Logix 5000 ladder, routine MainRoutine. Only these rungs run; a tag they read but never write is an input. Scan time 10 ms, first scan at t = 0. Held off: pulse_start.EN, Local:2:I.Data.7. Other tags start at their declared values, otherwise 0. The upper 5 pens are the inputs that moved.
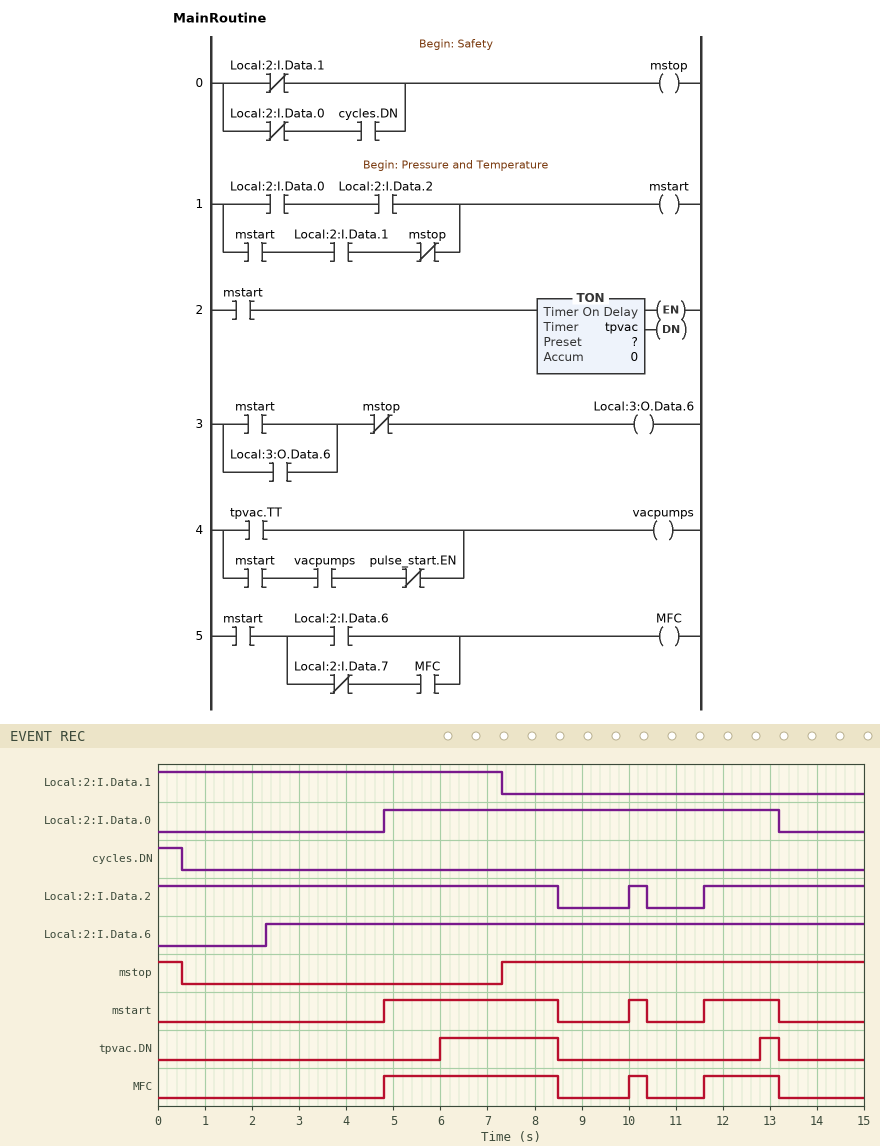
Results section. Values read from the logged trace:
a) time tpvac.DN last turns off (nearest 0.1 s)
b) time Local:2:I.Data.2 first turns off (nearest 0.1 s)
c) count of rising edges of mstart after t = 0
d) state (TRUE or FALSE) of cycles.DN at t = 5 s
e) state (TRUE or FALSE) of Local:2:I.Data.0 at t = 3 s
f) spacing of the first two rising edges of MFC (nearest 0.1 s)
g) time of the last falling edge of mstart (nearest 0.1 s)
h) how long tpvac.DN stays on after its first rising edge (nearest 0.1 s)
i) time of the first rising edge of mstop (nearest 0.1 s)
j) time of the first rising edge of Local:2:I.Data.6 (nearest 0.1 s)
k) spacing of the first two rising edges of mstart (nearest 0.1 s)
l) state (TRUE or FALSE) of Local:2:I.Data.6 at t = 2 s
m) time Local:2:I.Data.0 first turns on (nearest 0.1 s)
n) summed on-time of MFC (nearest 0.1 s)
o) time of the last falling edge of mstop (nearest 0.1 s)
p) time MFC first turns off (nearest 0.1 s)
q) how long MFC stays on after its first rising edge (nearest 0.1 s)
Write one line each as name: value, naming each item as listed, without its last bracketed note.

time tpvac.DN last turns off: 13.2 s
time Local:2:I.Data.2 first turns off: 8.5 s
count of rising edges of mstart after t = 0: 3
state (TRUE or FALSE) of cycles.DN at t = 5 s: FALSE
state (TRUE or FALSE) of Local:2:I.Data.0 at t = 3 s: FALSE
spacing of the first two rising edges of MFC: 5.2 s
time of the last falling edge of mstart: 13.2 s
how long tpvac.DN stays on after its first rising edge: 2.5 s
time of the first rising edge of mstop: 7.3 s
time of the first rising edge of Local:2:I.Data.6: 2.3 s
spacing of the first two rising edges of mstart: 5.2 s
state (TRUE or FALSE) of Local:2:I.Data.6 at t = 2 s: FALSE
time Local:2:I.Data.0 first turns on: 4.8 s
summed on-time of MFC: 5.7 s
time of the last falling edge of mstop: 0.5 s
time MFC first turns off: 8.5 s
how long MFC stays on after its first rising edge: 3.7 s
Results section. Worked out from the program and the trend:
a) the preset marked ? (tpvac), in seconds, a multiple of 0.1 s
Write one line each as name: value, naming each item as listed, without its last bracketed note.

the preset marked ? (tpvac), in seconds, a multiple of 0.1 s: 1.2 s
